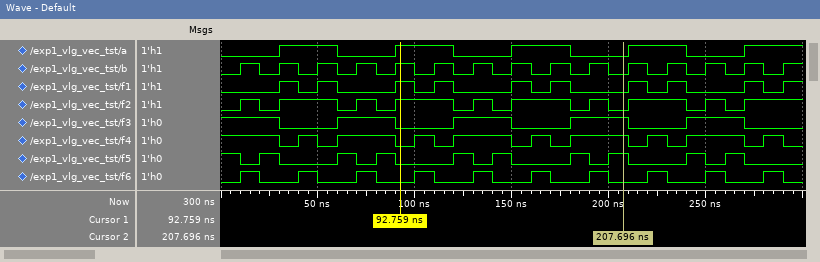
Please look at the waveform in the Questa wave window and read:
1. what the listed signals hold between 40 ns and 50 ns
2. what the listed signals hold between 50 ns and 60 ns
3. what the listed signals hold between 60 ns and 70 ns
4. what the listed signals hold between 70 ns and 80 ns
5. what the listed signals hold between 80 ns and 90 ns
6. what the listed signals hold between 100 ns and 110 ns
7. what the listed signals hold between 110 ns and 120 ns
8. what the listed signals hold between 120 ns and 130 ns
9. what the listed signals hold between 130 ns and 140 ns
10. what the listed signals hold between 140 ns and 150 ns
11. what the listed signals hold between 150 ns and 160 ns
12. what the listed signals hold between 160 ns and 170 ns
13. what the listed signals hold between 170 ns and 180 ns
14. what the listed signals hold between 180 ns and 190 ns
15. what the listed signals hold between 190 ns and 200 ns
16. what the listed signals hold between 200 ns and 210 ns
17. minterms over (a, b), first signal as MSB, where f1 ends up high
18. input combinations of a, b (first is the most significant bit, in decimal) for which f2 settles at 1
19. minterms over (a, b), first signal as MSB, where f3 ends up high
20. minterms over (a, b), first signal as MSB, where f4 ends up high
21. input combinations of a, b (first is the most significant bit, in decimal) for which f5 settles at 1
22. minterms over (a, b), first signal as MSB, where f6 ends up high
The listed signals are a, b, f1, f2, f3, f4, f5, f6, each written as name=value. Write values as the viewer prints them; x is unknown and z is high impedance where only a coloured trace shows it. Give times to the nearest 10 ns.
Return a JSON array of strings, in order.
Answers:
["a=1, b=0, f1=0, f2=1, f3=0, f4=1, f5=0, f6=1", "a=1, b=1, f1=1, f2=1, f3=0, f4=0, f5=0, f6=0", "a=0, b=0, f1=0, f2=0, f3=1, f4=1, f5=1, f6=0", "a=0, b=1, f1=0, f2=1, f3=1, f4=1, f5=0, f6=1", "a=0, b=0, f1=0, f2=0, f3=1, f4=1, f5=1, f6=0", "a=1, b=0, f1=0, f2=1, f3=0, f4=1, f5=0, f6=1", "a=1, b=1, f1=1, f2=1, f3=0, f4=0, f5=0, f6=0", "a=0, b=0, f1=0, f2=0, f3=1, f4=1, f5=1, f6=0", "a=0, b=1, f1=0, f2=1, f3=1, f4=1, f5=0, f6=1", "a=0, b=0, f1=0, f2=0, f3=1, f4=1, f5=1, f6=0", "a=1, b=1, f1=1, f2=1, f3=0, f4=0, f5=0, f6=0", "a=1, b=0, f1=0, f2=1, f3=0, f4=1, f5=0, f6=1", "a=1, b=1, f1=1, f2=1, f3=0, f4=0, f5=0, f6=0", "a=0, b=0, f1=0, f2=0, f3=1, f4=1, f5=1, f6=0", "a=0, b=1, f1=0, f2=1, f3=1, f4=1, f5=0, f6=1", "a=0, b=0, f1=0, f2=0, f3=1, f4=1, f5=1, f6=0", "3", "1, 2, 3", "0, 1", "0, 1, 2", "0", "1, 2"]
